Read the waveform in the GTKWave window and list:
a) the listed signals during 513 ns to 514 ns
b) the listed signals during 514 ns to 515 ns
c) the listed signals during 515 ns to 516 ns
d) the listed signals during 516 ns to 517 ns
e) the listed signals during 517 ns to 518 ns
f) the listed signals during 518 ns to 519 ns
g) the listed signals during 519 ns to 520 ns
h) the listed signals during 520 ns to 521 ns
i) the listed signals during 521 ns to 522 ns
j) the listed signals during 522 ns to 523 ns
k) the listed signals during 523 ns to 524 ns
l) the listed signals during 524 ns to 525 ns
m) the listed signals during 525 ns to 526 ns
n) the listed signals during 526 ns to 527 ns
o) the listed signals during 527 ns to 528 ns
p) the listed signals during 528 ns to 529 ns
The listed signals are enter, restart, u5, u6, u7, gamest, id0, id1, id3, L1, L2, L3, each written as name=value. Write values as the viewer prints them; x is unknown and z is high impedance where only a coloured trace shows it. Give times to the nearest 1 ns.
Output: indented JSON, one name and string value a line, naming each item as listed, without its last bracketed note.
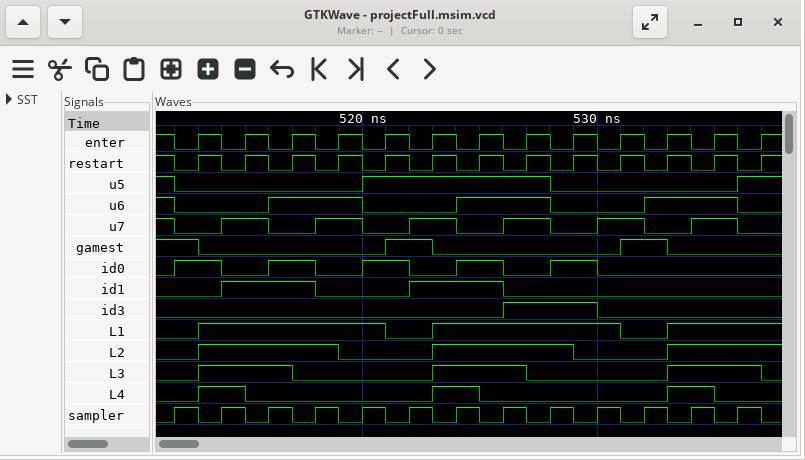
{
  "the listed signals during 513 ns to 514 ns": "enter=1, restart=1, u5=0, u6=0, u7=0, gamest=0, id0=1, id1=0, id3=0, L1=1, L2=1, L3=1",
  "the listed signals during 514 ns to 515 ns": "enter=0, restart=0, u5=0, u6=0, u7=1, gamest=0, id0=0, id1=1, id3=0, L1=1, L2=1, L3=1",
  "the listed signals during 515 ns to 516 ns": "enter=1, restart=1, u5=0, u6=0, u7=1, gamest=0, id0=0, id1=1, id3=0, L1=1, L2=1, L3=1",
  "the listed signals during 516 ns to 517 ns": "enter=0, restart=0, u5=0, u6=1, u7=0, gamest=0, id0=1, id1=1, id3=0, L1=1, L2=1, L3=1",
  "the listed signals during 517 ns to 518 ns": "enter=1, restart=1, u5=0, u6=1, u7=0, gamest=0, id0=1, id1=1, id3=0, L1=1, L2=1, L3=0",
  "the listed signals during 518 ns to 519 ns": "enter=0, restart=0, u5=0, u6=1, u7=1, gamest=0, id0=0, id1=0, id3=0, L1=1, L2=1, L3=0",
  "the listed signals during 519 ns to 520 ns": "enter=1, restart=1, u5=0, u6=1, u7=1, gamest=0, id0=0, id1=0, id3=0, L1=1, L2=0, L3=0",
  "the listed signals during 520 ns to 521 ns": "enter=0, restart=0, u5=1, u6=0, u7=0, gamest=0, id0=1, id1=0, id3=0, L1=1, L2=0, L3=0",
  "the listed signals during 521 ns to 522 ns": "enter=1, restart=1, u5=1, u6=0, u7=0, gamest=1, id0=1, id1=0, id3=0, L1=0, L2=0, L3=0",
  "the listed signals during 522 ns to 523 ns": "enter=0, restart=0, u5=1, u6=0, u7=1, gamest=1, id0=0, id1=1, id3=0, L1=0, L2=0, L3=0",
  "the listed signals during 523 ns to 524 ns": "enter=1, restart=1, u5=1, u6=0, u7=1, gamest=0, id0=0, id1=1, id3=0, L1=1, L2=1, L3=1",
  "the listed signals during 524 ns to 525 ns": "enter=0, restart=0, u5=1, u6=1, u7=0, gamest=0, id0=1, id1=1, id3=0, L1=1, L2=1, L3=1",
  "the listed signals during 525 ns to 526 ns": "enter=1, restart=1, u5=1, u6=1, u7=0, gamest=0, id0=1, id1=1, id3=0, L1=1, L2=1, L3=1",
  "the listed signals during 526 ns to 527 ns": "enter=0, restart=0, u5=1, u6=1, u7=1, gamest=0, id0=0, id1=0, id3=1, L1=1, L2=1, L3=1",
  "the listed signals during 527 ns to 528 ns": "enter=1, restart=1, u5=1, u6=1, u7=1, gamest=0, id0=0, id1=0, id3=1, L1=1, L2=1, L3=0",
  "the listed signals during 528 ns to 529 ns": "enter=0, restart=0, u5=0, u6=0, u7=0, gamest=0, id0=1, id1=0, id3=1, L1=1, L2=1, L3=0"
}
